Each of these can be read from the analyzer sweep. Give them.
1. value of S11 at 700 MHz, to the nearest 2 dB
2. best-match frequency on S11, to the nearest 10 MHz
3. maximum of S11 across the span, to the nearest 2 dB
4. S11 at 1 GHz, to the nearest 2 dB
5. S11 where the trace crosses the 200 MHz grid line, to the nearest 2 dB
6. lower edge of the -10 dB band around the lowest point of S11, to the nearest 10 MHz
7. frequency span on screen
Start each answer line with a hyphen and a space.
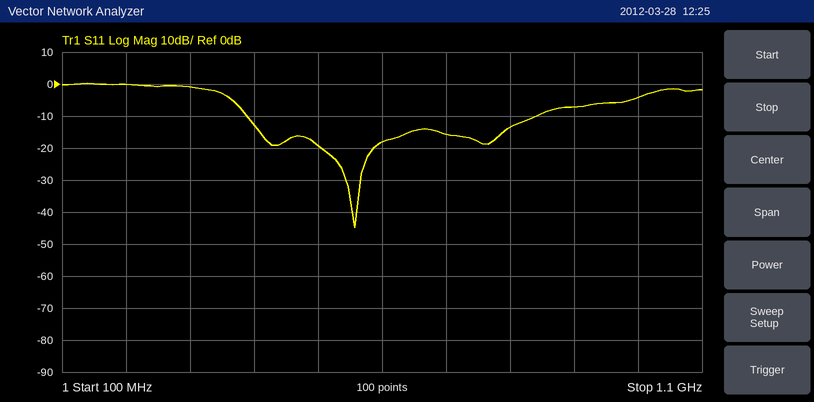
- -16 dB
- 560 MHz
- 0 dB
- -4 dB
- 0 dB
- 390 MHz
- 1 GHz
